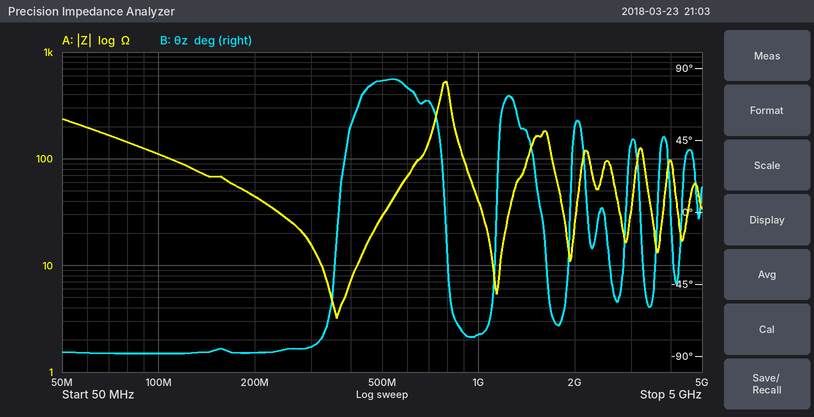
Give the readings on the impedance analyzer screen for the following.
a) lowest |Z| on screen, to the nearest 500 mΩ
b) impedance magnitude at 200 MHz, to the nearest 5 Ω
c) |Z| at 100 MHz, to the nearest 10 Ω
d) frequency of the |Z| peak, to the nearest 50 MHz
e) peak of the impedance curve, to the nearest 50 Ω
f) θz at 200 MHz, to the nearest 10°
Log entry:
3.0 Ω
45 Ω
110 Ω
800 MHz
550 Ω
-90°
